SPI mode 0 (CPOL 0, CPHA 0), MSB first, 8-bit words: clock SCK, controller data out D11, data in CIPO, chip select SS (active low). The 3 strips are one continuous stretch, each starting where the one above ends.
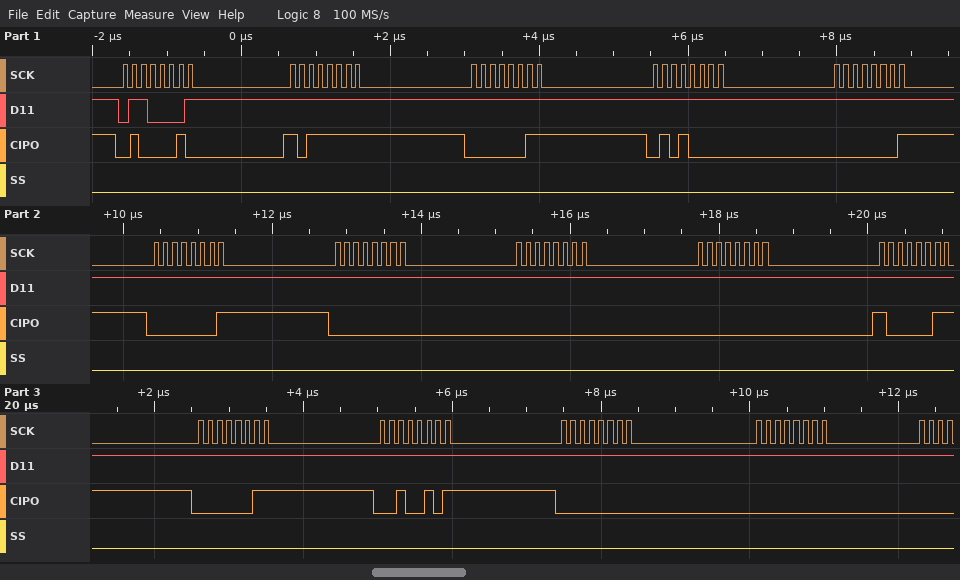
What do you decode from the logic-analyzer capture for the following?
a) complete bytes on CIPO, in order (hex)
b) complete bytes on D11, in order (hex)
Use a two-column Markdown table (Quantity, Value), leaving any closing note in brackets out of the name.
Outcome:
| Quantity | Value |
|---|---|
| complete bytes on CIPO, in order | 42 BF 03 50 01 01 00 00 00 83 03 25 00 00 |
| complete bytes on D11, in order | 61 FF FF FF FF FF FF FF FF FF FF FF FF FF |
